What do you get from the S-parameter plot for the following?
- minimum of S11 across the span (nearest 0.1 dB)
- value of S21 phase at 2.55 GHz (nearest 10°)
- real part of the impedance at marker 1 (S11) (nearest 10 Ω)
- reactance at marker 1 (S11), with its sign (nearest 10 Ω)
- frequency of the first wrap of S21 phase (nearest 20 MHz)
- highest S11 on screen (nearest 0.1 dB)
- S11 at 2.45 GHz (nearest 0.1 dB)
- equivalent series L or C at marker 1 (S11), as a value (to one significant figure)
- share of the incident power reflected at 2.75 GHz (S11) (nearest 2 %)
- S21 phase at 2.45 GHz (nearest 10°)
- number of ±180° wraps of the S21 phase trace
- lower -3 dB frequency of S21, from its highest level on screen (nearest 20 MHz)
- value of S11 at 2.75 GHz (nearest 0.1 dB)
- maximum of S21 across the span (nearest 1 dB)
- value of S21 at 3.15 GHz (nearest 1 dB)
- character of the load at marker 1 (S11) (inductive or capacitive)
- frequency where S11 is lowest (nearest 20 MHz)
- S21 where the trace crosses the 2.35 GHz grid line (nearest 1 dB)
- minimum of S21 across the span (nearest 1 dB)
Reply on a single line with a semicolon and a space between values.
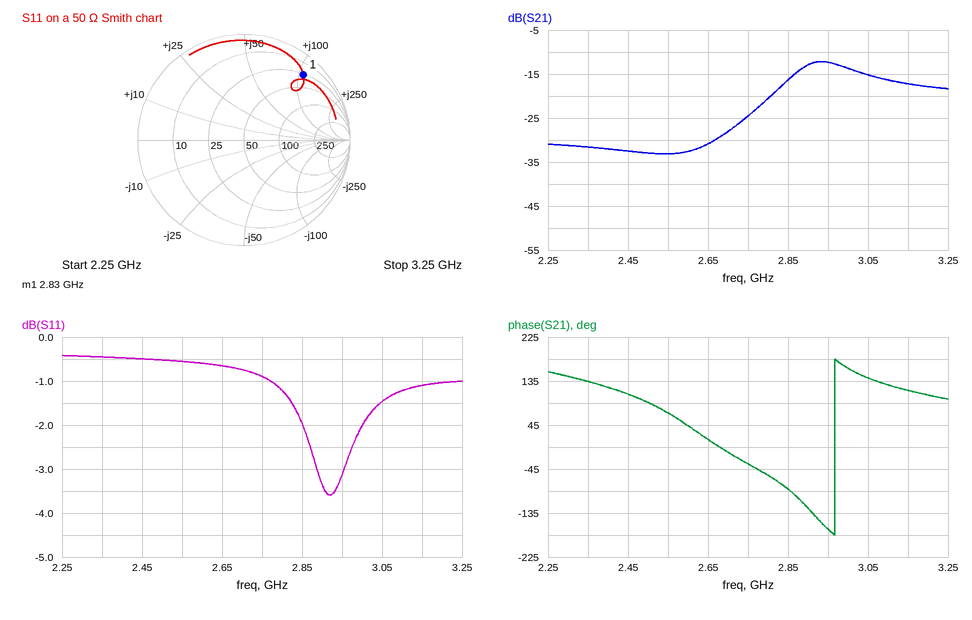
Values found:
-3.6 dB; 70°; 30 Ω; +110 Ω; 2.96 GHz; -0.4 dB; -0.5 dB; 6 nH; 82 %; 110°; 1; 2.86 GHz; -0.9 dB; -12 dB; -17 dB; inductive; 2.92 GHz; -32 dB; -33 dB
